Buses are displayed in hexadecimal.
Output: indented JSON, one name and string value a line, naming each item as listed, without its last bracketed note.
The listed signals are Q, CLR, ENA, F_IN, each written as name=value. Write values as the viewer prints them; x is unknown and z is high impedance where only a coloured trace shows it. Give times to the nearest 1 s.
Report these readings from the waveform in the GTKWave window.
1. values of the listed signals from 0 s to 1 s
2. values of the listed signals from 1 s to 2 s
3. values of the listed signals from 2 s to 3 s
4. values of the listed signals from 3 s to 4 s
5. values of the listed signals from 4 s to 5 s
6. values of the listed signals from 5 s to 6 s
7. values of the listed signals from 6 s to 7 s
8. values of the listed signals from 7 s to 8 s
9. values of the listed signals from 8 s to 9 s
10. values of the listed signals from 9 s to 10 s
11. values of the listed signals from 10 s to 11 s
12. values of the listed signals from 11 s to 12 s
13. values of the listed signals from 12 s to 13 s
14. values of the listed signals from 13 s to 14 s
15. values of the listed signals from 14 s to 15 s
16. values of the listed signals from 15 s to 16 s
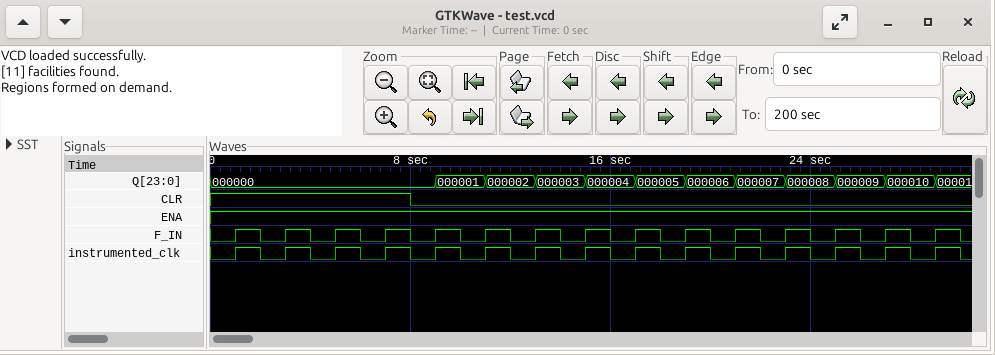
{
  "values of the listed signals from 0 s to 1 s": "Q=000000, CLR=1, ENA=1, F_IN=0",
  "values of the listed signals from 1 s to 2 s": "Q=000000, CLR=1, ENA=1, F_IN=1",
  "values of the listed signals from 2 s to 3 s": "Q=000000, CLR=1, ENA=1, F_IN=0",
  "values of the listed signals from 3 s to 4 s": "Q=000000, CLR=1, ENA=1, F_IN=1",
  "values of the listed signals from 4 s to 5 s": "Q=000000, CLR=1, ENA=1, F_IN=0",
  "values of the listed signals from 5 s to 6 s": "Q=000000, CLR=1, ENA=1, F_IN=1",
  "values of the listed signals from 6 s to 7 s": "Q=000000, CLR=1, ENA=1, F_IN=0",
  "values of the listed signals from 7 s to 8 s": "Q=000000, CLR=1, ENA=1, F_IN=1",
  "values of the listed signals from 8 s to 9 s": "Q=000000, CLR=0, ENA=1, F_IN=0",
  "values of the listed signals from 9 s to 10 s": "Q=000001, CLR=0, ENA=1, F_IN=1",
  "values of the listed signals from 10 s to 11 s": "Q=000001, CLR=0, ENA=1, F_IN=0",
  "values of the listed signals from 11 s to 12 s": "Q=000002, CLR=0, ENA=1, F_IN=1",
  "values of the listed signals from 12 s to 13 s": "Q=000002, CLR=0, ENA=1, F_IN=0",
  "values of the listed signals from 13 s to 14 s": "Q=000003, CLR=0, ENA=1, F_IN=1",
  "values of the listed signals from 14 s to 15 s": "Q=000003, CLR=0, ENA=1, F_IN=0",
  "values of the listed signals from 15 s to 16 s": "Q=000004, CLR=0, ENA=1, F_IN=1"
}
